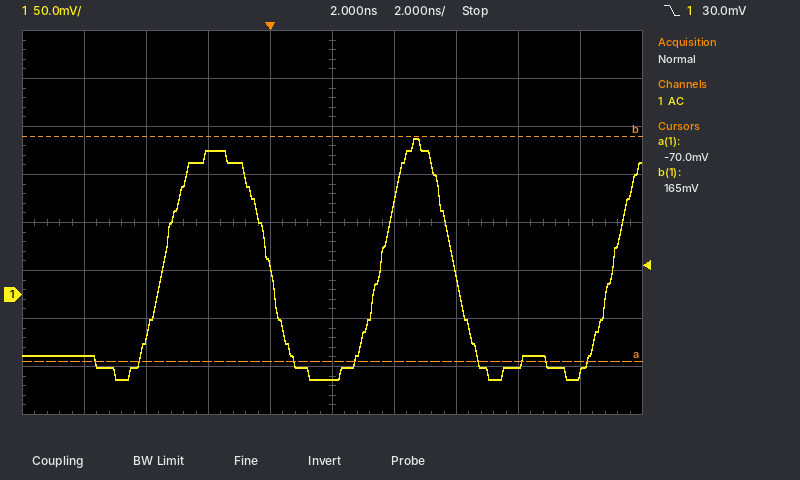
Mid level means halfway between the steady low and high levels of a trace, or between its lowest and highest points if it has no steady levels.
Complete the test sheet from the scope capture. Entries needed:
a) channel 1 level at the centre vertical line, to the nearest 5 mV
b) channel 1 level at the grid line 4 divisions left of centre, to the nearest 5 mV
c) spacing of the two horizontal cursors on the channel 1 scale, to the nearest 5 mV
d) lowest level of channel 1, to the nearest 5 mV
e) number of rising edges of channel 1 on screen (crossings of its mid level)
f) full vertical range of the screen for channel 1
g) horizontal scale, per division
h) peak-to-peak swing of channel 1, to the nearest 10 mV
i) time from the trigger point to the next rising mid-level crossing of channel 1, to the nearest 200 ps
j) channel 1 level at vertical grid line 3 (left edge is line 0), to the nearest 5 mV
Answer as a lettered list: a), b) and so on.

a) -90 mV
b) -65 mV
c) 235 mV
d) -90 mV
e) 3
f) 400 mV
g) 2 ns
h) 250 mV
i) 3.6 ns
j) 150 mV
